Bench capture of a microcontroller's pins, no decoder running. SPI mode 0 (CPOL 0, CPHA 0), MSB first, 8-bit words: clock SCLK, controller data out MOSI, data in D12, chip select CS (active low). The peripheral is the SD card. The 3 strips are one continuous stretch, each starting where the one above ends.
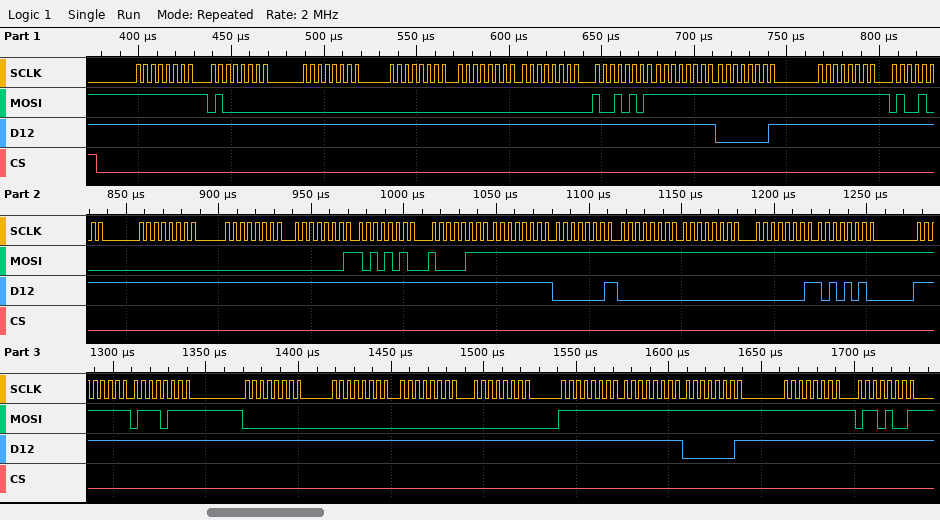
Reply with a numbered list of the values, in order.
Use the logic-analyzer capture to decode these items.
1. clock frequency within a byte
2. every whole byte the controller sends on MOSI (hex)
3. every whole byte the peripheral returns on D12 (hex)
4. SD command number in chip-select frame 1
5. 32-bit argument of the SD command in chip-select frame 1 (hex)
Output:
1. 250 kHz
2. FF 40 00 00 00 00 95 FF FF FF 48 00 00 01 AA 87 FF FF FF FF FF FF FF 77 00 00 00 00 FF FF FF FF 69
3. FF FF FF FF FF FF FF FF 01 FF FF FF FF FF FF FF FF 01 00 00 01 AA FF FF FF FF FF FF FF FF 01 FF FF
4. CMD0
5. 0x00000000
